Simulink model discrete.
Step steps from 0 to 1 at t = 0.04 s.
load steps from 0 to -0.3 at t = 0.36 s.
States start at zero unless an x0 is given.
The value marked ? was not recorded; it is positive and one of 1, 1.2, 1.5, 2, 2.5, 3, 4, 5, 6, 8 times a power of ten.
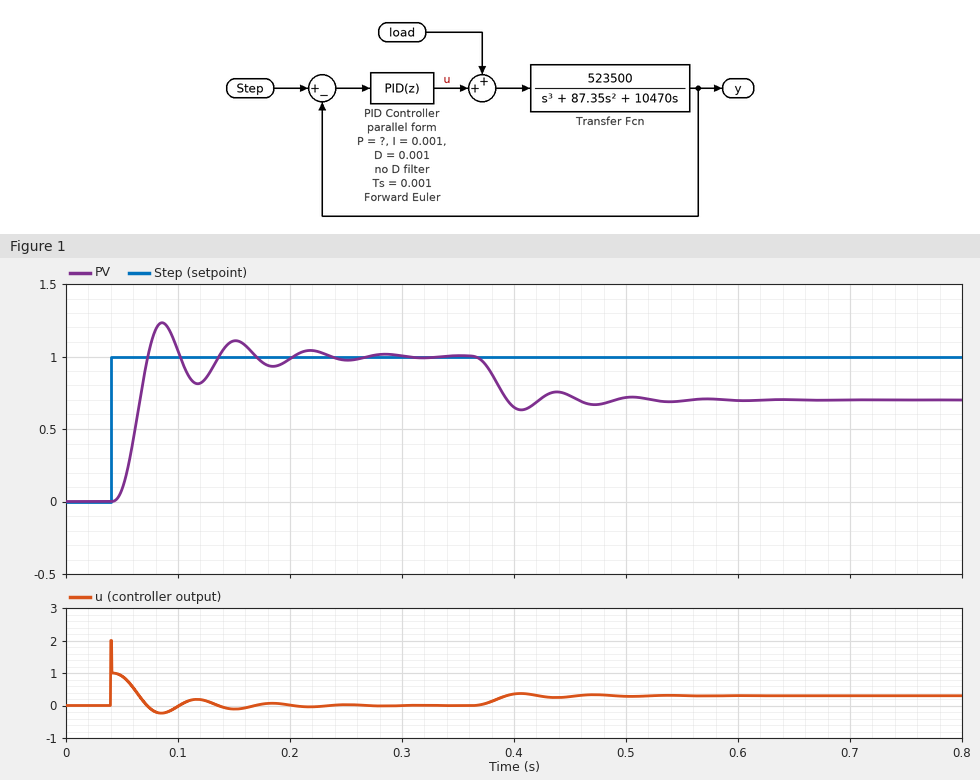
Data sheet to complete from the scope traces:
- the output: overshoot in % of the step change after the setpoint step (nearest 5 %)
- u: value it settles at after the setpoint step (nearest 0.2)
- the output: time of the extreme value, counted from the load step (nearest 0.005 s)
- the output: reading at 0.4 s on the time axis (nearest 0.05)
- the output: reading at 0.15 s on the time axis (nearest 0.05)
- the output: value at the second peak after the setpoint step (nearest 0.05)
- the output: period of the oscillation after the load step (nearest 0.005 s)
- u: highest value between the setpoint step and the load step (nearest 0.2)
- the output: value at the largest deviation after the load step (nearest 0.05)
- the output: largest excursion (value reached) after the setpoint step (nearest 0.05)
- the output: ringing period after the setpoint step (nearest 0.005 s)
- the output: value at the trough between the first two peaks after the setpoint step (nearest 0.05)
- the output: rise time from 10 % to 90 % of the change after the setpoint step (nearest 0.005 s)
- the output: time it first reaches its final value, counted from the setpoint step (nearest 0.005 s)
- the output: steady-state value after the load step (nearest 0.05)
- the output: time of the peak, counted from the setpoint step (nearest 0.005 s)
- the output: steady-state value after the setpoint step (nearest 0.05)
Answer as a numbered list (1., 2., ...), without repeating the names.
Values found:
1. 25 %
2. 0.0
3. 0.045 s
4. 0.65
5. 1.10
6. 1.10
7. 0.065 s
8. 2.0
9. 0.65
10. 1.25
11. 0.065 s
12. 0.80
13. 0.020 s
14. 0.035 s
15. 0.70
16. 0.045 s
17. 1.00
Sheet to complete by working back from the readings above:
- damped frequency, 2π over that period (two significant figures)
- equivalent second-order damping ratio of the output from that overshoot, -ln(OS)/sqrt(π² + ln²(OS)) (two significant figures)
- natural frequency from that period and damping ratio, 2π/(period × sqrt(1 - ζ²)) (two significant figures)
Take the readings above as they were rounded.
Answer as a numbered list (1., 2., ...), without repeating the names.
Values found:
1. 97 rad/s
2. 0.40
3. 110 rad/s
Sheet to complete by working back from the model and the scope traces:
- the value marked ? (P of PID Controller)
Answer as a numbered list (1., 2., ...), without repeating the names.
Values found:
1. 1
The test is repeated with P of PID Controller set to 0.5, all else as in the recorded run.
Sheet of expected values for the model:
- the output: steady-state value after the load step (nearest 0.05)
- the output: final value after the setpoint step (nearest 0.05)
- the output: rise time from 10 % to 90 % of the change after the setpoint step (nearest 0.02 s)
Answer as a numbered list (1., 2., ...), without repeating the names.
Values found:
1. 0.40
2. 1.00
3. 0.08 s
